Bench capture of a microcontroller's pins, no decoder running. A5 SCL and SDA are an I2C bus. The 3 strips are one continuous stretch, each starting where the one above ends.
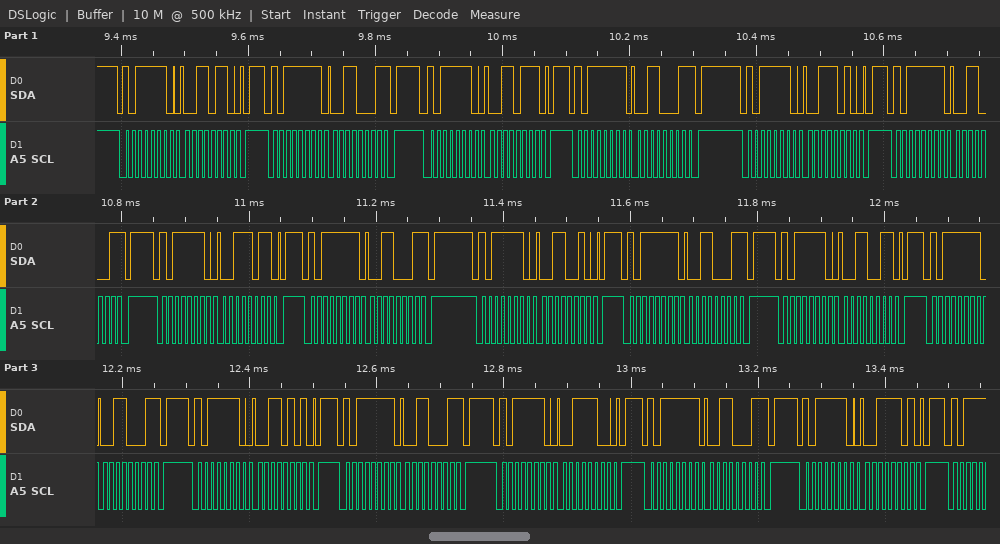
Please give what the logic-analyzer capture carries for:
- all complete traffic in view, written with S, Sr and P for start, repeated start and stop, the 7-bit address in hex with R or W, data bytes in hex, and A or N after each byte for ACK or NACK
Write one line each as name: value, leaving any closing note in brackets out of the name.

all complete traffic in view, written with S, Sr and P for start, repeated start and stop, the 7-bit address in hex with R or W, data bytes in hex, and A or N after each byte for ACK or NACK: S 5FW A 36 A P S 5FR A 31 N P S 5FW A 37 A P S 5FR A 31 N P S 5FW A 3A A P S 5FR A 31 N P S 5FW A 3B A P S 5FR A 31 N P S 5FW A 32 A P S 5FR A 31 N P S 5FW A 33 A P S 5FR A 31 N P S 5FW A 35 A P S 5FR A 31 N P S 5FW A 3C A P S 5FR A 31 N P S 5FW A 3D A P
